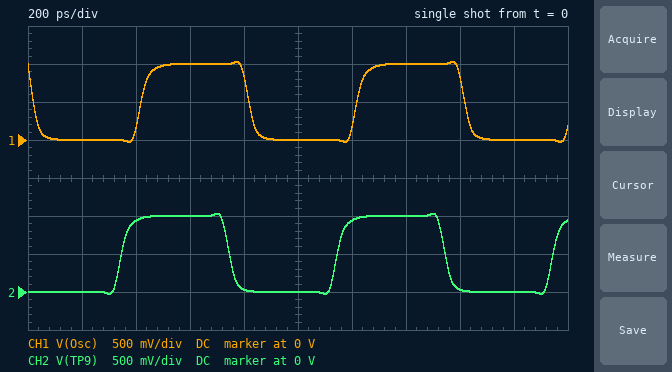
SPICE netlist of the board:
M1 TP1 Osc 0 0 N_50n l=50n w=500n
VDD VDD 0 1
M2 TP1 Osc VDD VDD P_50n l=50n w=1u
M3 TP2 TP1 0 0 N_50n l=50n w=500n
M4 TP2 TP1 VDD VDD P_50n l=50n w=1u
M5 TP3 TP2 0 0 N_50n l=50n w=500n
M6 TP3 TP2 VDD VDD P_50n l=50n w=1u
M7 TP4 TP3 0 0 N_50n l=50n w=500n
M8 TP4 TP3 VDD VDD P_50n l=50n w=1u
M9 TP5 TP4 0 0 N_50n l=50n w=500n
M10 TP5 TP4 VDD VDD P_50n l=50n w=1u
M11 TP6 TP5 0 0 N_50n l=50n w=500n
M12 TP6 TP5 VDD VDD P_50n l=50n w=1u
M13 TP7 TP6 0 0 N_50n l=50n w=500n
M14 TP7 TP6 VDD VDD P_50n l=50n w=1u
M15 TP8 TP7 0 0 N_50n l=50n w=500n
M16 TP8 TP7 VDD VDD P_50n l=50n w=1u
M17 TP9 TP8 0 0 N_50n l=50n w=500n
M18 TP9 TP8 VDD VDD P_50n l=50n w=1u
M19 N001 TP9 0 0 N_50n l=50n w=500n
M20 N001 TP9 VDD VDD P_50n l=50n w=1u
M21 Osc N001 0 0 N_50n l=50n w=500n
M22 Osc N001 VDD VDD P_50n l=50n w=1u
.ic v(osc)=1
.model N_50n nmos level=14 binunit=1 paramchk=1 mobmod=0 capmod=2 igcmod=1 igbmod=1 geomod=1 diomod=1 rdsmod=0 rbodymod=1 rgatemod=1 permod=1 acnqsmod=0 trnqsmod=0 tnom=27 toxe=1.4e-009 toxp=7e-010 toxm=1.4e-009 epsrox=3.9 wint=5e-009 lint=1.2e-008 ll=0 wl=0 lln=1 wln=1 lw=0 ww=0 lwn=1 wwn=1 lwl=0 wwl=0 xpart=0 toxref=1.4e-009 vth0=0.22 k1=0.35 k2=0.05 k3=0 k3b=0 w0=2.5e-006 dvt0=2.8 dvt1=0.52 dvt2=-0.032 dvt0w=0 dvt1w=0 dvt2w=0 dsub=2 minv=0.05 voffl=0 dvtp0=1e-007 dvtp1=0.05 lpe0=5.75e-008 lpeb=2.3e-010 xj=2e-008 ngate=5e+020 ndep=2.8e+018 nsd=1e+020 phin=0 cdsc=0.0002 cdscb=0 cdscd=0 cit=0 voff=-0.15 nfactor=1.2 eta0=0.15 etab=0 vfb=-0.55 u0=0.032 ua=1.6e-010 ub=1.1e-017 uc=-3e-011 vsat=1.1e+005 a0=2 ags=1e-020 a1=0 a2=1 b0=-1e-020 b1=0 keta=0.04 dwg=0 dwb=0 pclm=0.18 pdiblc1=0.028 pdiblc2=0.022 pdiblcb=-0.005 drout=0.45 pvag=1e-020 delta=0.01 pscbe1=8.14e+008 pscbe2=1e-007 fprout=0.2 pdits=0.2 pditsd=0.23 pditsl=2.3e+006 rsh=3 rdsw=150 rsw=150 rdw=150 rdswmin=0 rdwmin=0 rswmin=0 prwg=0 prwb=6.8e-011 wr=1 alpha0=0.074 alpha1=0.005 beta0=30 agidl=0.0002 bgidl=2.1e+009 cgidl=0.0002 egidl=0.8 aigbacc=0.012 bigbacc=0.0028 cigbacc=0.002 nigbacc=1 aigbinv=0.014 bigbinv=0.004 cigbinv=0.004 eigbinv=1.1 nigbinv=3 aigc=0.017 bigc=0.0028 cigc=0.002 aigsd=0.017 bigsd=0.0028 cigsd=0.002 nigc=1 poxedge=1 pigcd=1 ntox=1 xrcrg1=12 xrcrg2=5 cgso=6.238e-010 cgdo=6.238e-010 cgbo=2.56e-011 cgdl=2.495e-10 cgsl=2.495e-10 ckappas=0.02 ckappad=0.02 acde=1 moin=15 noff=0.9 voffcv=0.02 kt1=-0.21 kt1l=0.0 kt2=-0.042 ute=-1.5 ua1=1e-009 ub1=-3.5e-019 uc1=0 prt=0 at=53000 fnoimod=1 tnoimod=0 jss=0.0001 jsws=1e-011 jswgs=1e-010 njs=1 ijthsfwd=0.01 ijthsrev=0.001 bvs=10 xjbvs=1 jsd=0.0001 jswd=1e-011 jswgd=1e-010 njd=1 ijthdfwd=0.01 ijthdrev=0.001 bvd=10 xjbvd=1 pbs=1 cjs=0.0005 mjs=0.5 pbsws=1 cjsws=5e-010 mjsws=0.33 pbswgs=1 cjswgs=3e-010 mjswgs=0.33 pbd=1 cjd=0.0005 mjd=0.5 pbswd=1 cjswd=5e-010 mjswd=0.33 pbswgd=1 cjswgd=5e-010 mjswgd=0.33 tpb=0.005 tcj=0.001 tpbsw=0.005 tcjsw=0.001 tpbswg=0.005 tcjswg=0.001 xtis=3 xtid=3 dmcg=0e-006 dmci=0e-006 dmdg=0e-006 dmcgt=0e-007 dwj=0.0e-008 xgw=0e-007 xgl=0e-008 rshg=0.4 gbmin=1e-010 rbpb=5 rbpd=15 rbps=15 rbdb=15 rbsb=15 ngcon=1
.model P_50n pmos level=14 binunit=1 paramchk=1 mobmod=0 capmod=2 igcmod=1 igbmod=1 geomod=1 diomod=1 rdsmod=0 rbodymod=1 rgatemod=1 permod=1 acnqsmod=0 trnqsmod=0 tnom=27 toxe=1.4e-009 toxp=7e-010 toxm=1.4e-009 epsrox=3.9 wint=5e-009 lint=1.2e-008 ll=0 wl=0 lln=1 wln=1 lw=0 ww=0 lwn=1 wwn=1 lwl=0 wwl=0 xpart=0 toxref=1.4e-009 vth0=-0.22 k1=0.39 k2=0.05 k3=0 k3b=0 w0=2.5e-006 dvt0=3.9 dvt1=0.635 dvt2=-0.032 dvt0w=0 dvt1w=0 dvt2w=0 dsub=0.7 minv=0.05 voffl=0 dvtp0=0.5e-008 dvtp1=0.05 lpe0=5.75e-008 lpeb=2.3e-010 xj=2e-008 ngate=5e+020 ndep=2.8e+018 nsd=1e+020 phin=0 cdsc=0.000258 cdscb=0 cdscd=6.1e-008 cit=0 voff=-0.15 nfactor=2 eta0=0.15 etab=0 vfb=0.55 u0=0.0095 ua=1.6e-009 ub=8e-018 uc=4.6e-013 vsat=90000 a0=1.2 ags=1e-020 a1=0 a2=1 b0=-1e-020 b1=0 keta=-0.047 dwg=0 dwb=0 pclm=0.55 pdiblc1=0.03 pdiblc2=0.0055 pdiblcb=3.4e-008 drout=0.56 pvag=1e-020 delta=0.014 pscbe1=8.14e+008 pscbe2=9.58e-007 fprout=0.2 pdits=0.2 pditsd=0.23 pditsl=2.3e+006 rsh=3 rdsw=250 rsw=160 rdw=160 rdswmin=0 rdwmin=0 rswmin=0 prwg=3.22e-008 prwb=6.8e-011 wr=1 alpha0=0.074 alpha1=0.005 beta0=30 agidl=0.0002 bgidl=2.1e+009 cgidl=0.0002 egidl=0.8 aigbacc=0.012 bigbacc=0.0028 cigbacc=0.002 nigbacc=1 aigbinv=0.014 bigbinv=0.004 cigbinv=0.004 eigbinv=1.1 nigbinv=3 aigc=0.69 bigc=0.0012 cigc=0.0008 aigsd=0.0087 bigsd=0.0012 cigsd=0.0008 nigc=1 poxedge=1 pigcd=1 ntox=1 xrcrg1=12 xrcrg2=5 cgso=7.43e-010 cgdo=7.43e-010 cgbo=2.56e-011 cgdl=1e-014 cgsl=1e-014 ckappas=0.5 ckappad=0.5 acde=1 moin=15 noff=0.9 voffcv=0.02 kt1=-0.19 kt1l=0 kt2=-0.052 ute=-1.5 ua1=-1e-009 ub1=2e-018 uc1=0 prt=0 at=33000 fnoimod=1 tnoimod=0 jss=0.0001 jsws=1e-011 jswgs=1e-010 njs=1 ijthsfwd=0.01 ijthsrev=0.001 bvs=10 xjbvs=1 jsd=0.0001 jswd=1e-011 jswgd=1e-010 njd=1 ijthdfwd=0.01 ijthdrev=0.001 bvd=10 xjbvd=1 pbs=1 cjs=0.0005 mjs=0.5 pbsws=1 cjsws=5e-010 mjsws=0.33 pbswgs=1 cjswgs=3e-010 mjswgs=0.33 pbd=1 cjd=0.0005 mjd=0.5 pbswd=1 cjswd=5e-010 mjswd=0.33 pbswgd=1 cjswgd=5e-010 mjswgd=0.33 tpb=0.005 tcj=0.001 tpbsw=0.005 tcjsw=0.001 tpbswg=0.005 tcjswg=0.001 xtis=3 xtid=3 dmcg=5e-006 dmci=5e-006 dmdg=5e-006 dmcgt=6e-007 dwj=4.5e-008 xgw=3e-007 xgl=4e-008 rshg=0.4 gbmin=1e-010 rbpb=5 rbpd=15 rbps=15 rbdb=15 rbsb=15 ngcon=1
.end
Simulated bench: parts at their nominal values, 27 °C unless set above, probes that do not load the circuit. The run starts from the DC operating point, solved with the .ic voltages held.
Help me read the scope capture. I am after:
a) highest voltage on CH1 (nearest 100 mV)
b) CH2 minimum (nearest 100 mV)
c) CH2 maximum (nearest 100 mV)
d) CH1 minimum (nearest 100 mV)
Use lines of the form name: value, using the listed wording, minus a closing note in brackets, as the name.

highest voltage on CH1: 1.0 V
CH2 minimum: 0 V
CH2 maximum: 1.0 V
CH1 minimum: 0 V
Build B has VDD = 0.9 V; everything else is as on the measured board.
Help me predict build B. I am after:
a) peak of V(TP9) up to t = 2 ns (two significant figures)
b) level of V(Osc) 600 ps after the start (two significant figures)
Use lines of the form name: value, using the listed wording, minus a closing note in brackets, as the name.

peak of V(TP9) up to t = 2 ns: 930 mV
level of V(Osc) 600 ps after the start: 900 mV
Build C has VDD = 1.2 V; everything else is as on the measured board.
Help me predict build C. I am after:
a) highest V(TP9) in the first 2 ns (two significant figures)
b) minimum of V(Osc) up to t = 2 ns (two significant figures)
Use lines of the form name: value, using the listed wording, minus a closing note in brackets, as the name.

highest V(TP9) in the first 2 ns: 1.2 V
minimum of V(Osc) up to t = 2 ns: -25 mV
